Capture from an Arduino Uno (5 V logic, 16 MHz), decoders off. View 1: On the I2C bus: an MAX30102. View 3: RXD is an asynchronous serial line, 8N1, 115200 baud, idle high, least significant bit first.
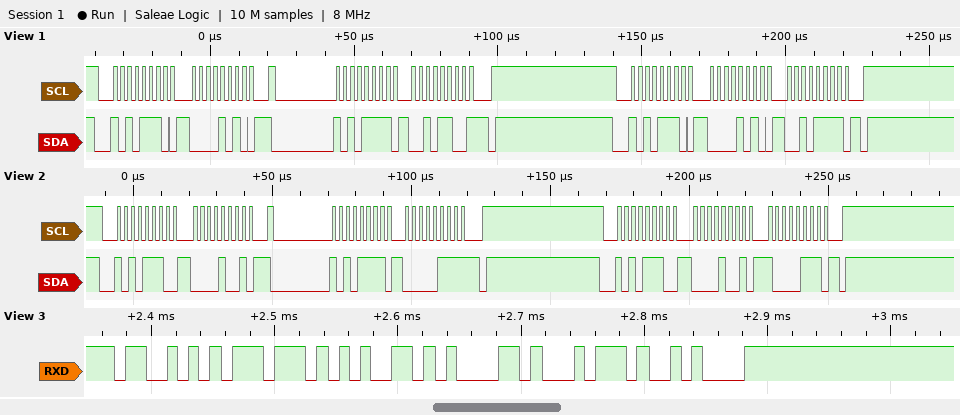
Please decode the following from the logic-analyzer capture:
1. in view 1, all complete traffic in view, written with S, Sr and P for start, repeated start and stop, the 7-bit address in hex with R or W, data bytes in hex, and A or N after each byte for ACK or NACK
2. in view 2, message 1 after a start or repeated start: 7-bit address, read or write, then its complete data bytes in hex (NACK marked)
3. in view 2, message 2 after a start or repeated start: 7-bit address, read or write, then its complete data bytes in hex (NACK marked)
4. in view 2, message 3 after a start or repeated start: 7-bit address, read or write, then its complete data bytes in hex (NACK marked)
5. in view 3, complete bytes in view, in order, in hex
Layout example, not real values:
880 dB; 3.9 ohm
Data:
S 57W A 0A A Sr 57R A 2C N P S 57W A 0A A 2F A P; 0x57 write: 09; 0x57 read: 07 NACK; 0x57 write: 09 87; 53 77 65 61 74 0A
